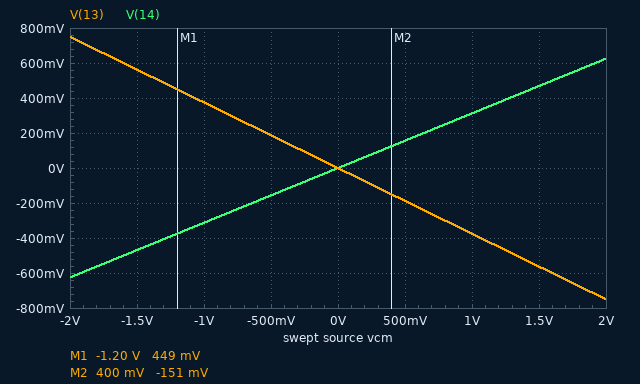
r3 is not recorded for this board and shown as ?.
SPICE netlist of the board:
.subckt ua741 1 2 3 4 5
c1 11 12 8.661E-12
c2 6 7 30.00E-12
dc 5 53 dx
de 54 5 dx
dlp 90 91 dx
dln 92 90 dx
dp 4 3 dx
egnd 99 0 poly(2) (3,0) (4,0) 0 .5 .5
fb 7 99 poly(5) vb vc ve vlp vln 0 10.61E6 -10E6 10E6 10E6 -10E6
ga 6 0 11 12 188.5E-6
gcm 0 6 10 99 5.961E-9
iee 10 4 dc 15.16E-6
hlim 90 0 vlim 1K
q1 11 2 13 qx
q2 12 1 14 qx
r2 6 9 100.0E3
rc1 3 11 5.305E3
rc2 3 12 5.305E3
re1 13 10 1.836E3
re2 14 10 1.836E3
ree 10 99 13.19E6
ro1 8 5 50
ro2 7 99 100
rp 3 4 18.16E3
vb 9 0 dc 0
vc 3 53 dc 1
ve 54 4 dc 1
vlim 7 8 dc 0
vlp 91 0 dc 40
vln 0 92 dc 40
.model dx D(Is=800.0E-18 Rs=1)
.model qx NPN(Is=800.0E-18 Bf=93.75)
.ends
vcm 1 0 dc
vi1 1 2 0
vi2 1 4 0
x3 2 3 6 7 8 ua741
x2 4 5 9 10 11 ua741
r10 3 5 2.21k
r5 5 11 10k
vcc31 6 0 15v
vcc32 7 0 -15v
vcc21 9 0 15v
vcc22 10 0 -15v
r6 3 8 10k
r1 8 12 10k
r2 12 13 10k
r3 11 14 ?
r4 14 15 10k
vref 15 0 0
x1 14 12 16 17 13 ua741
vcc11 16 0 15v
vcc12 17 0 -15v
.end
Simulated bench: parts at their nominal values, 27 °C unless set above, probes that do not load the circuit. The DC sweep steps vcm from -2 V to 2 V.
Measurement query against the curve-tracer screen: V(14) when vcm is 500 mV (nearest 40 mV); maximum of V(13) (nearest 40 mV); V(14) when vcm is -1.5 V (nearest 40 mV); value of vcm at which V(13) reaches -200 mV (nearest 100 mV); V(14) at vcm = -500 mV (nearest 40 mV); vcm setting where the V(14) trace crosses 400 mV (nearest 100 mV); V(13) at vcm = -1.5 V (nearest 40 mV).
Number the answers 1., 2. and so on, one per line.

1. 160 mV
2. 760 mV
3. -480 mV
4. 500 mV
5. -160 mV
6. 1.3 V
7. 560 mV
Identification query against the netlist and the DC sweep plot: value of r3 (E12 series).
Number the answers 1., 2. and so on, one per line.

1. 22 kΩ
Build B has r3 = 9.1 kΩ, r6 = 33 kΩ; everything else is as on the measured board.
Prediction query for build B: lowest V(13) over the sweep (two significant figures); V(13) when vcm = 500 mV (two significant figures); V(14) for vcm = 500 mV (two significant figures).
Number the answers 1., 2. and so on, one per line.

1. -96 mV
2. 22 mV
3. 260 mV
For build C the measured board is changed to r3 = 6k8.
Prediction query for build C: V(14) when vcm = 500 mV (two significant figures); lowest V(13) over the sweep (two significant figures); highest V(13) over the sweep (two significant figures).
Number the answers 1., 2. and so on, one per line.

1. 300 mV
2. -380 mV
3. 380 mV
